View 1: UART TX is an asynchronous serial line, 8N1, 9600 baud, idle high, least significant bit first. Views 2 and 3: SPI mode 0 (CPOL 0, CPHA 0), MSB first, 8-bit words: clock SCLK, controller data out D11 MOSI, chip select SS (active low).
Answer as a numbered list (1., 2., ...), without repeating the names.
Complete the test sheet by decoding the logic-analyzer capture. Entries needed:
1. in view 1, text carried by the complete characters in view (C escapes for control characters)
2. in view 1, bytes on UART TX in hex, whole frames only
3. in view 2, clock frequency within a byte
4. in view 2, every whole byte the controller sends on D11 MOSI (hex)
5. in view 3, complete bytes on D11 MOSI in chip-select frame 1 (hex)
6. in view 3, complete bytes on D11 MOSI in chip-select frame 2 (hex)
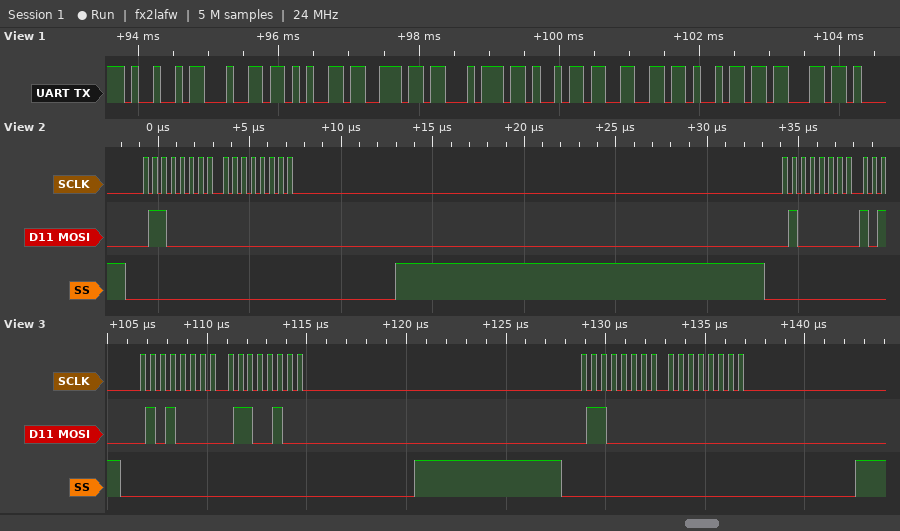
1. "Identific"
2. 49 64 65 6E 74 69 66 69 63
3. 2 MHz
4. 60 00 40
5. 0x50 0x64
6. 0x60 0x00
